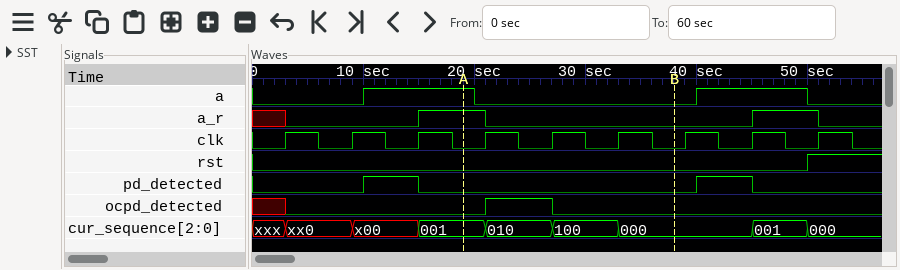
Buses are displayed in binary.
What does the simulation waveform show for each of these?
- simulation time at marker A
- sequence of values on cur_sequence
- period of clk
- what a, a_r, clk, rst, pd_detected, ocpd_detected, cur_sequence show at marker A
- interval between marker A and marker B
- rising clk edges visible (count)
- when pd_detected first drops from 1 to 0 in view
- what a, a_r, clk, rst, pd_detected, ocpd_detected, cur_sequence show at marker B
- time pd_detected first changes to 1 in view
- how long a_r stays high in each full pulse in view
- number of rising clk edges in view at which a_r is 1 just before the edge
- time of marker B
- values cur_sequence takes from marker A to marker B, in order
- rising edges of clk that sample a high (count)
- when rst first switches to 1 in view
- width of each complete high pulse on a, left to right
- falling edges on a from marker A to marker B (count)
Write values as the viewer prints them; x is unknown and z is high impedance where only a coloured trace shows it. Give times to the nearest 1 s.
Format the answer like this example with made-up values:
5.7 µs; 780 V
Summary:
19 s; xxx, xx0, x00, 001, 010, 100, 000, 001, 000; 6 s; a=1, a_r=1, clk=0, rst=0, pd_detected=0, ocpd_detected=0, cur_sequence=001; 19 s; 9; 15 s; a=0, a_r=0, clk=0, rst=0, pd_detected=0, ocpd_detected=0, cur_sequence=000; 10 s; 6 s, 6 s; 2; 38 s; 001, 010, 100, 000; 2; 50 s; 10 s, 10 s; 1
